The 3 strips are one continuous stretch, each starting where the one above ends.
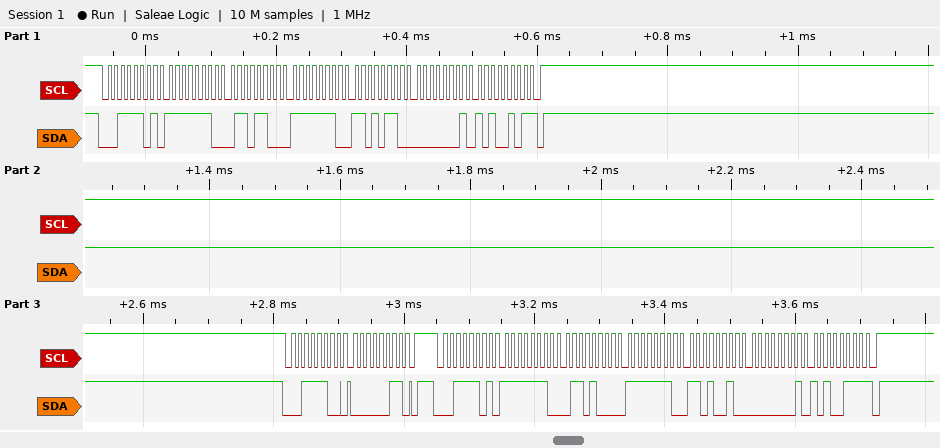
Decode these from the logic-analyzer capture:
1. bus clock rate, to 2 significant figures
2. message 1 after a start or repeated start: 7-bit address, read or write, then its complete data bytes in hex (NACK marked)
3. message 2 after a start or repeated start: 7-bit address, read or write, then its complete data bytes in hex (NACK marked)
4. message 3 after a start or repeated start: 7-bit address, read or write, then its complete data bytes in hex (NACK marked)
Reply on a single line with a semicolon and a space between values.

100 kHz; 0x1E read: FE 6C FE D6 01 A5 NACK; 0x1E write: 03; 0x1E read: FE 68 FE D2 01 A7 NACK
